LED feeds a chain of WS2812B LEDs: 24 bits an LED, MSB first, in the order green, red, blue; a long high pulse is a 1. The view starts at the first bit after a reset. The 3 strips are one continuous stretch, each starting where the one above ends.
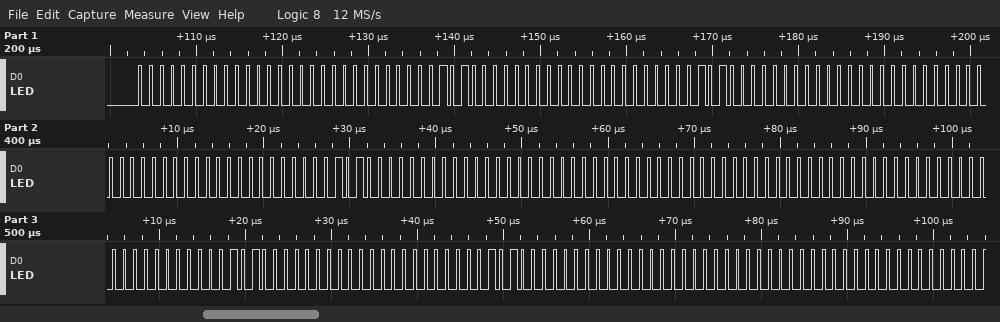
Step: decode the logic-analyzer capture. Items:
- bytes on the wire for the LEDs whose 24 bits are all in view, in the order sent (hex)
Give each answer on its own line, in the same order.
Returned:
00 00 00 0A 00 00 0A 00 00 00 00 00 0A 00 00 00 00 00 00 00 00 0A 00 00 0A 00 00 00 00 00
